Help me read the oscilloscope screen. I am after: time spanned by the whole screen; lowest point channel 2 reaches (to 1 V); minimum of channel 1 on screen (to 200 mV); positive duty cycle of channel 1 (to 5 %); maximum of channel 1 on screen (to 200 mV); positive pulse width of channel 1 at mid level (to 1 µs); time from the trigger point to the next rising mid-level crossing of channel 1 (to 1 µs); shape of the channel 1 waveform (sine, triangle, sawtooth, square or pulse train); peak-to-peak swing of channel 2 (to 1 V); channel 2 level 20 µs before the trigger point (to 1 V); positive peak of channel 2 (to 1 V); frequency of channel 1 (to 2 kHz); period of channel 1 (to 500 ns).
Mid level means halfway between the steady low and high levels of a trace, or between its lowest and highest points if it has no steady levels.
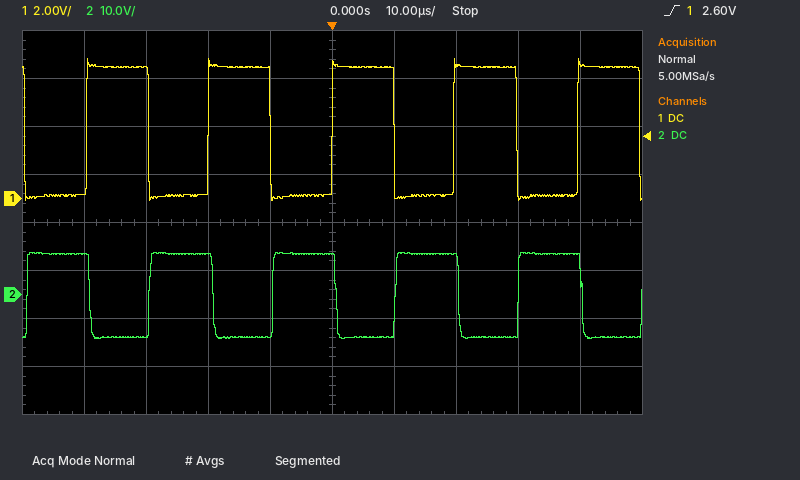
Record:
100 µs
-9 V
0.0 V
50 %
5.8 V
10 µs
20 µs
square
18 V
8 V
9 V
50 kHz
20.0 µs
